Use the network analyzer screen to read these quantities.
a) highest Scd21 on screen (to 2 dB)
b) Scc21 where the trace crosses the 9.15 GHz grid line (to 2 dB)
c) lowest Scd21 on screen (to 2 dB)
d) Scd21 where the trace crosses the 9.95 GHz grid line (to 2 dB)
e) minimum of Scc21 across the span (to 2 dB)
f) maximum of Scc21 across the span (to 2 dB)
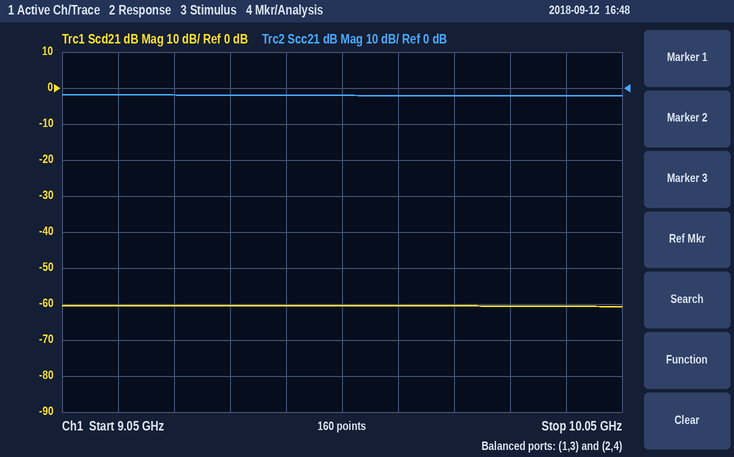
-60 dB
-2 dB
-60 dB
-60 dB
-2 dB
-2 dB
